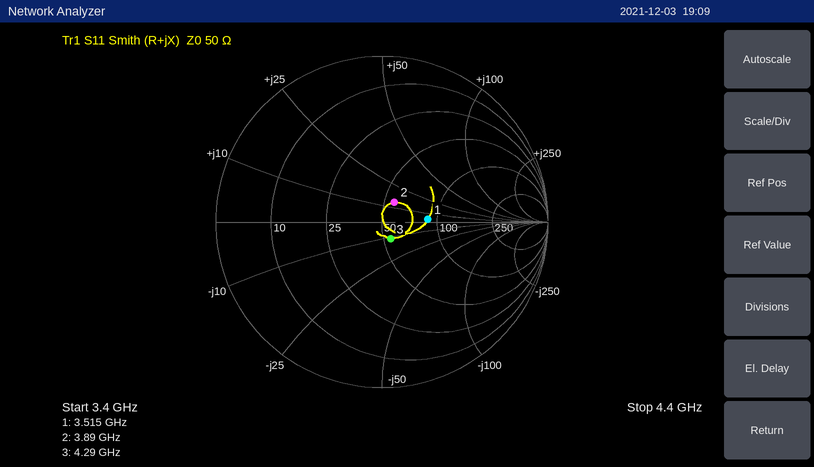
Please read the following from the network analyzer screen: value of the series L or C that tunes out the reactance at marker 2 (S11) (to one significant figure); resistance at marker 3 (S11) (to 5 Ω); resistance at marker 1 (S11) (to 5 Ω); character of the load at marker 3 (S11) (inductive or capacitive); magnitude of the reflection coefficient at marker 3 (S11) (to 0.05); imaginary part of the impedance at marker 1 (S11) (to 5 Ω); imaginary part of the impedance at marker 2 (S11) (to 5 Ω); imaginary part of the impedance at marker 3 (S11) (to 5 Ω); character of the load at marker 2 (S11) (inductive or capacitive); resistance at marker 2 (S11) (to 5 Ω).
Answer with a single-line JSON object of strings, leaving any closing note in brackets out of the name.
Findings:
{"value of the series L or C that tunes out the reactance at marker 2 (S11)": "3 pF", "resistance at marker 3 (S11)": "55 Ω", "resistance at marker 1 (S11)": "90 Ω", "character of the load at marker 3 (S11)": "capacitive", "magnitude of the reflection coefficient at marker 3 (S11)": "0.10", "imaginary part of the impedance at marker 1 (S11)": "+5 Ω", "imaginary part of the impedance at marker 2 (S11)": "+15 Ω", "imaginary part of the impedance at marker 3 (S11)": "-10 Ω", "character of the load at marker 2 (S11)": "inductive", "resistance at marker 2 (S11)": "55 Ω"}
